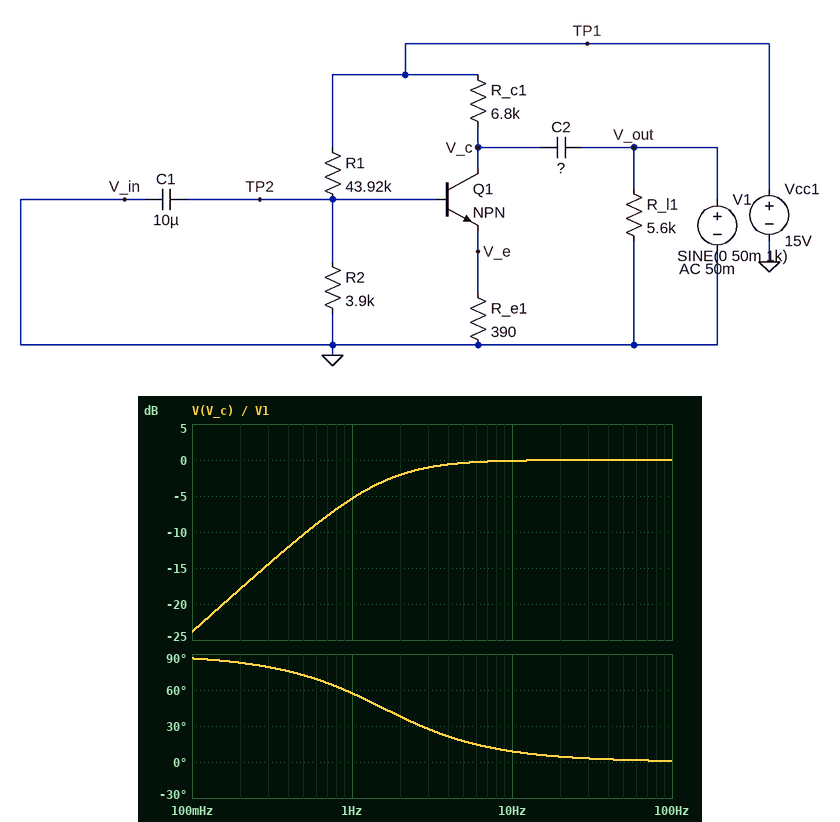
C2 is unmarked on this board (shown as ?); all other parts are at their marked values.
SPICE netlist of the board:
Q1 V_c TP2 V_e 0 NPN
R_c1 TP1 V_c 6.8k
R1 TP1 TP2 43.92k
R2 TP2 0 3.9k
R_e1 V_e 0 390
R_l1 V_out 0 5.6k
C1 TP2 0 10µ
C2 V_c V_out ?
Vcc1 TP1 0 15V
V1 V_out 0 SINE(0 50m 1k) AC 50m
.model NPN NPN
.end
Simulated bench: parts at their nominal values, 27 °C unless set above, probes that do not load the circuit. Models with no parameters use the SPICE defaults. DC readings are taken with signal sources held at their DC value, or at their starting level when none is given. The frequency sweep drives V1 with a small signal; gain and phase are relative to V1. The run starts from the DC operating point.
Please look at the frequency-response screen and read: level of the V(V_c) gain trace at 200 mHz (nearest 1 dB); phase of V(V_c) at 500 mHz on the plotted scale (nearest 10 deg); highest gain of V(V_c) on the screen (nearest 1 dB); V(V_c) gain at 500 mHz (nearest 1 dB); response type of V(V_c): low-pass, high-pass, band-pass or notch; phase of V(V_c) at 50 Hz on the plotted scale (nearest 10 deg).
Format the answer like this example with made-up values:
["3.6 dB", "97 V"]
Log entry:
["-18 dB", "70 deg", "0 dB", "-10 dB", "high-pass", "0 deg"]
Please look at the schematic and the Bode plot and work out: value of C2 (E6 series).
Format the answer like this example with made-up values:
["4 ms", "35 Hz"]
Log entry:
["15 µF"]
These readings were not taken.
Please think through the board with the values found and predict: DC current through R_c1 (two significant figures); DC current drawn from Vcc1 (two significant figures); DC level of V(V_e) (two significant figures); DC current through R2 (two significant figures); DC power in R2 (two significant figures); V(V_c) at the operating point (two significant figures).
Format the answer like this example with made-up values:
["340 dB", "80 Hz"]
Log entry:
["1.0 mA", "1.4 mA", "410 mV", "300 µA", "360 µW", "7.9 V"]
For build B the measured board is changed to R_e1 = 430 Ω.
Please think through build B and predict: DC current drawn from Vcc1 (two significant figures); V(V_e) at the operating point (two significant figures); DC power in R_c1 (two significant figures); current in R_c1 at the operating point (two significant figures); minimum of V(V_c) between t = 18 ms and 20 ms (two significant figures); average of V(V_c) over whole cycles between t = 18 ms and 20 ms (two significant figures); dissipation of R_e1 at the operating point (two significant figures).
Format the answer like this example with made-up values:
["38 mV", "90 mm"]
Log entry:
["1.3 mA", "420 mV", "6.2 mW", "960 µA", "8.4 V", "8.5 V", "400 µW"]
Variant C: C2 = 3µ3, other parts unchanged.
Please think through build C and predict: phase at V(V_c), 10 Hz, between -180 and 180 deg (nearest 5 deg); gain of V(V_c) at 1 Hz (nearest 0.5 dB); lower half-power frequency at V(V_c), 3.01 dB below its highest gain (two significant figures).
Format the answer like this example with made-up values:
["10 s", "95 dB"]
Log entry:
["35 deg", "-17.0 dB", "7.1 Hz"]
